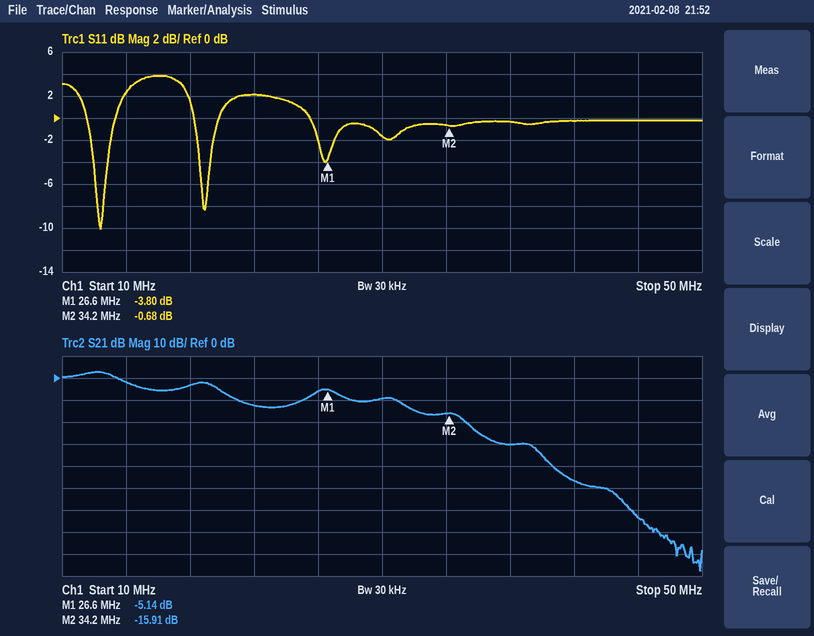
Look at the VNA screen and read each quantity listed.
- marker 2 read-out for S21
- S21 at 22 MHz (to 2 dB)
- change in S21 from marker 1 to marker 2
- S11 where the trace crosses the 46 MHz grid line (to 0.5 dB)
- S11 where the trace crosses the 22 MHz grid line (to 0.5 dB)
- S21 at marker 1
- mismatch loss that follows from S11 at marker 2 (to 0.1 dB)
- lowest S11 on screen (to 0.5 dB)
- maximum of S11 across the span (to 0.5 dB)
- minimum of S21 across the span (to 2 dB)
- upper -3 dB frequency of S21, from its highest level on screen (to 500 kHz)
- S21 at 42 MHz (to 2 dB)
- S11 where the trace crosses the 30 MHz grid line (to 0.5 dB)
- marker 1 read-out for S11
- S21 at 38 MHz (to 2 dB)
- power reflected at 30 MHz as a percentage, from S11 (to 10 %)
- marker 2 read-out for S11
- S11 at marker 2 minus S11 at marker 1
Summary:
-15.91 dB
-12 dB
-10.77 dB
0.0 dB
2.0 dB
-5.14 dB
8.4 dB
-10.0 dB
4.0 dB
-88 dB
13.5 MHz
-46 dB
-1.5 dB
-3.80 dB
-30 dB
70 %
-0.68 dB
3.12 dB
